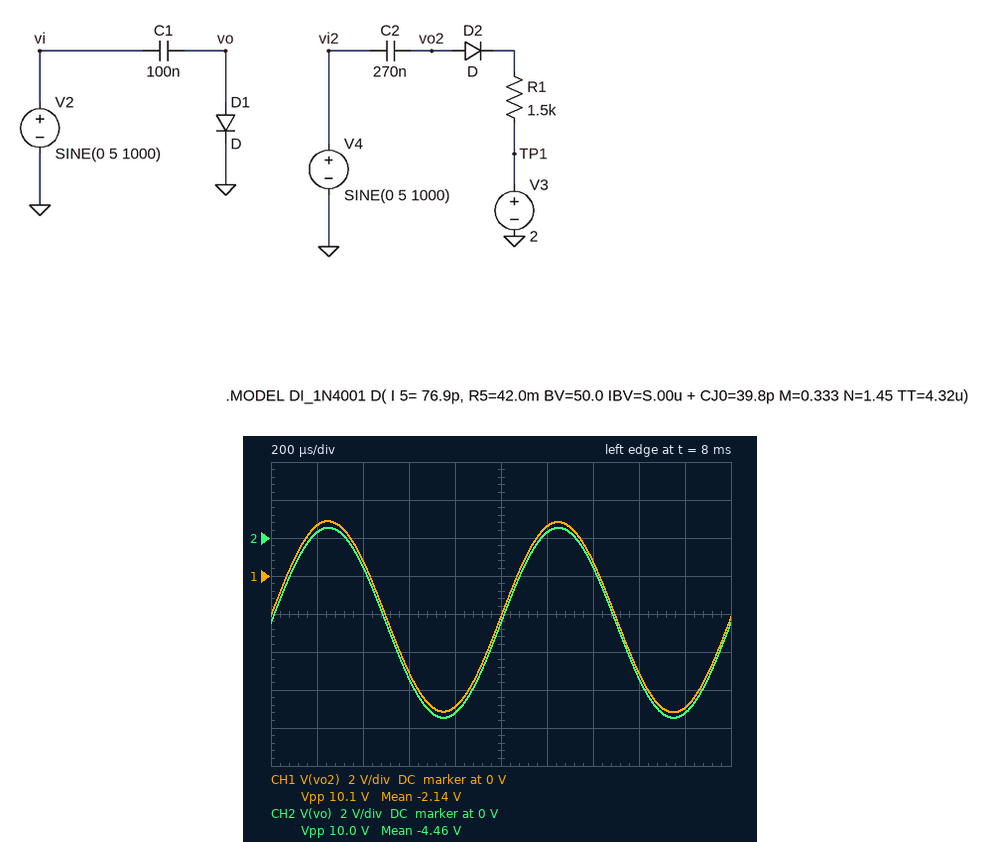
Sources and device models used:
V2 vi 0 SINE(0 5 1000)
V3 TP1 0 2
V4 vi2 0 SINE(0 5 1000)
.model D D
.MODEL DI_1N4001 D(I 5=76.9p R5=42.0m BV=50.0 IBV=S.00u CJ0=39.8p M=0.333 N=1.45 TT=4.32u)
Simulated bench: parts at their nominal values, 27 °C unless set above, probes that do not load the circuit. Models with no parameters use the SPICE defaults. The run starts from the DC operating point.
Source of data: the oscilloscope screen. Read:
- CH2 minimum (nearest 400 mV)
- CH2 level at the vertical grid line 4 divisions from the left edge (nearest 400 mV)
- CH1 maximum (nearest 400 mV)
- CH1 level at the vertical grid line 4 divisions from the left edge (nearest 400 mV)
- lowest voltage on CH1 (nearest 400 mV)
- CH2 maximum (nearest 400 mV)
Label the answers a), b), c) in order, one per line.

a) -9.6 V
b) -9.2 V
c) 2.8 V
d) -6.8 V
e) -7.2 V
f) 400 mV
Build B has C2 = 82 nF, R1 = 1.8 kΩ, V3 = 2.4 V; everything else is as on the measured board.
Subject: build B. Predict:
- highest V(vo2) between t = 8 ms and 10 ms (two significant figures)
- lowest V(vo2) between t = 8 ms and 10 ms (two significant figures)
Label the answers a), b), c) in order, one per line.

a) 3.0 V
b) -7.0 V
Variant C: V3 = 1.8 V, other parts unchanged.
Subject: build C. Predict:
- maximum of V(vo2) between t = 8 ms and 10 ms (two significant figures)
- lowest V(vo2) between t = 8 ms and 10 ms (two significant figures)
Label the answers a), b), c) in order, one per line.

a) 2.7 V
b) -7.4 V
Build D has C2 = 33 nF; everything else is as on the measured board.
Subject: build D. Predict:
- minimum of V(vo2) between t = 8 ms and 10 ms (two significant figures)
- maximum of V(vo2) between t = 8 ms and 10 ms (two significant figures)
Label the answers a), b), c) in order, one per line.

a) -7.5 V
b) 2.5 V
